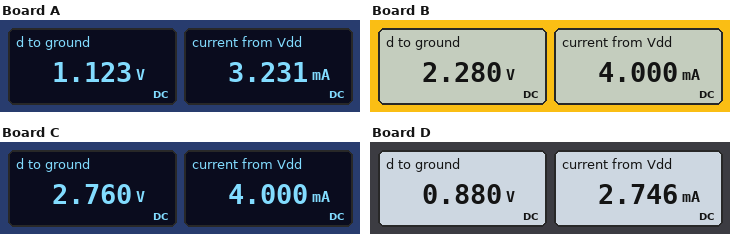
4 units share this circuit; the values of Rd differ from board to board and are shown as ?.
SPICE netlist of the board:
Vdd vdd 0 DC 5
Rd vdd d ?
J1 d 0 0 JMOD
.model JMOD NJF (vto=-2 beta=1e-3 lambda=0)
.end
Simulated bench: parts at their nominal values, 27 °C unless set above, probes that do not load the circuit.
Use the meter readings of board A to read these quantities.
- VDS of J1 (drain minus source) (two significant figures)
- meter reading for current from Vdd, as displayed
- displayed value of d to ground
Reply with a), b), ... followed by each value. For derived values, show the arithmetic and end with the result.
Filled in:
a) 1.123 V = 1.1 V
b) 3.231 mA
c) 1.123 V
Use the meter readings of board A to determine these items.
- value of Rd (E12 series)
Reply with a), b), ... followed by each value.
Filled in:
a) 1.2 kΩ
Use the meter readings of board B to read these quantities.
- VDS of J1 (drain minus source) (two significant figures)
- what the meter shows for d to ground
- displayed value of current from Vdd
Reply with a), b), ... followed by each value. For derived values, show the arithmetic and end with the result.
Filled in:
a) 2.28 V = 2.3 V
b) 2.280 V
c) 4.000 mA
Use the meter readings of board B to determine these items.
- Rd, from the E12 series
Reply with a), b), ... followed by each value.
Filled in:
a) 680 Ω
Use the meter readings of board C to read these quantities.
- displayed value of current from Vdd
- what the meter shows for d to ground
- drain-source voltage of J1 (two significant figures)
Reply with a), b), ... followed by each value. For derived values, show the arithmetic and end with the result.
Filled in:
a) 4.000 mA
b) 2.760 V
c) 2.76 V = 2.8 V
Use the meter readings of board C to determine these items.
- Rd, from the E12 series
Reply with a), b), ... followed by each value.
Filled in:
a) 560 Ω
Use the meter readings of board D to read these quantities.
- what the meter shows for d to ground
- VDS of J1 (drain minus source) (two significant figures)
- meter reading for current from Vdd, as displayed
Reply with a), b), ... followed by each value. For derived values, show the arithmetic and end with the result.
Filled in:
a) 0.880 V
b) 880 mV = 880 mV
c) 2.746 mA
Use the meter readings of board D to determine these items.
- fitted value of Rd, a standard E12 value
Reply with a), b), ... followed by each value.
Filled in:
a) 1.5 kΩ
